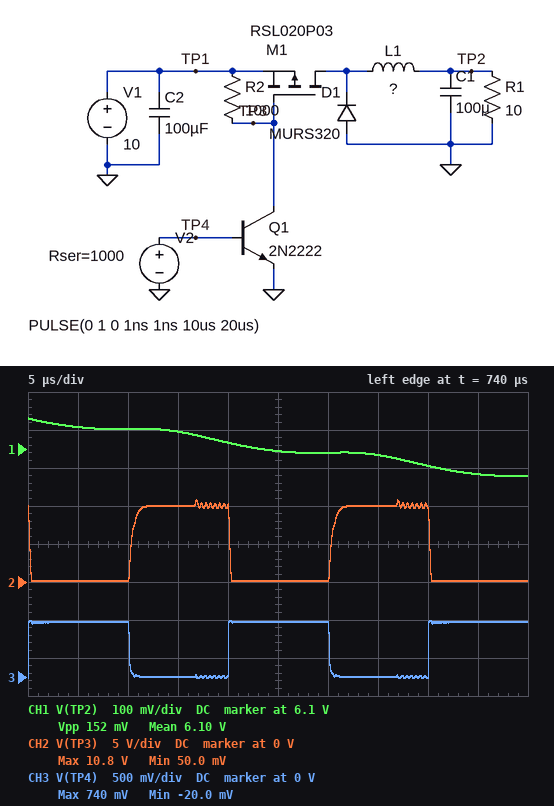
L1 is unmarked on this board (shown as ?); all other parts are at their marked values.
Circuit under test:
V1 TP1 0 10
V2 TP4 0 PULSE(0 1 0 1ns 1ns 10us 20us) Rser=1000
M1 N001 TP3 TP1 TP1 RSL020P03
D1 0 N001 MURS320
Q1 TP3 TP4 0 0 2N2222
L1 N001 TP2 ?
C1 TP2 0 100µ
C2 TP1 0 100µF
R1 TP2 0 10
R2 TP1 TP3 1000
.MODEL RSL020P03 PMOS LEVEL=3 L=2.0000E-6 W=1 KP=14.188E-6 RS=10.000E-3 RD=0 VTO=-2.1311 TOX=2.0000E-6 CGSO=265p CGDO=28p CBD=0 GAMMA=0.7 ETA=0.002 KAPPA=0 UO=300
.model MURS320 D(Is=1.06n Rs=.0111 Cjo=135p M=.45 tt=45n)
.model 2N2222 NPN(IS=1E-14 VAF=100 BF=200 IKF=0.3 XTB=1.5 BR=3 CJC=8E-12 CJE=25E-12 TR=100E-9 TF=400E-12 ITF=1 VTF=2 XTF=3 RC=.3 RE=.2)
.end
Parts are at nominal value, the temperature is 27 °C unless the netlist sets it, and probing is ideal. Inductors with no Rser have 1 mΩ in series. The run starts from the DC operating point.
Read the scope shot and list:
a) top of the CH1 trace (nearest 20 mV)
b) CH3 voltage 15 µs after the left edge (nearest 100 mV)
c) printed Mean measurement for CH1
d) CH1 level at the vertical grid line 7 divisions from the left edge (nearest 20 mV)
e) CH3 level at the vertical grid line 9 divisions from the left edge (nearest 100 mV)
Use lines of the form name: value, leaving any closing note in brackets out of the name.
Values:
top of the CH1 trace: 6.18 V
CH3 voltage 15 µs after the left edge: 0 V
printed Mean measurement for CH1: 6.10 V
CH1 level at the vertical grid line 7 divisions from the left edge: 6.08 V
CH3 level at the vertical grid line 9 divisions from the left edge: 700 mV
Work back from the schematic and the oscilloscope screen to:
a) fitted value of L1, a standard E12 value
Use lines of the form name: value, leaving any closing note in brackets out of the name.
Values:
fitted value of L1, a standard E12 value: 56 µH
